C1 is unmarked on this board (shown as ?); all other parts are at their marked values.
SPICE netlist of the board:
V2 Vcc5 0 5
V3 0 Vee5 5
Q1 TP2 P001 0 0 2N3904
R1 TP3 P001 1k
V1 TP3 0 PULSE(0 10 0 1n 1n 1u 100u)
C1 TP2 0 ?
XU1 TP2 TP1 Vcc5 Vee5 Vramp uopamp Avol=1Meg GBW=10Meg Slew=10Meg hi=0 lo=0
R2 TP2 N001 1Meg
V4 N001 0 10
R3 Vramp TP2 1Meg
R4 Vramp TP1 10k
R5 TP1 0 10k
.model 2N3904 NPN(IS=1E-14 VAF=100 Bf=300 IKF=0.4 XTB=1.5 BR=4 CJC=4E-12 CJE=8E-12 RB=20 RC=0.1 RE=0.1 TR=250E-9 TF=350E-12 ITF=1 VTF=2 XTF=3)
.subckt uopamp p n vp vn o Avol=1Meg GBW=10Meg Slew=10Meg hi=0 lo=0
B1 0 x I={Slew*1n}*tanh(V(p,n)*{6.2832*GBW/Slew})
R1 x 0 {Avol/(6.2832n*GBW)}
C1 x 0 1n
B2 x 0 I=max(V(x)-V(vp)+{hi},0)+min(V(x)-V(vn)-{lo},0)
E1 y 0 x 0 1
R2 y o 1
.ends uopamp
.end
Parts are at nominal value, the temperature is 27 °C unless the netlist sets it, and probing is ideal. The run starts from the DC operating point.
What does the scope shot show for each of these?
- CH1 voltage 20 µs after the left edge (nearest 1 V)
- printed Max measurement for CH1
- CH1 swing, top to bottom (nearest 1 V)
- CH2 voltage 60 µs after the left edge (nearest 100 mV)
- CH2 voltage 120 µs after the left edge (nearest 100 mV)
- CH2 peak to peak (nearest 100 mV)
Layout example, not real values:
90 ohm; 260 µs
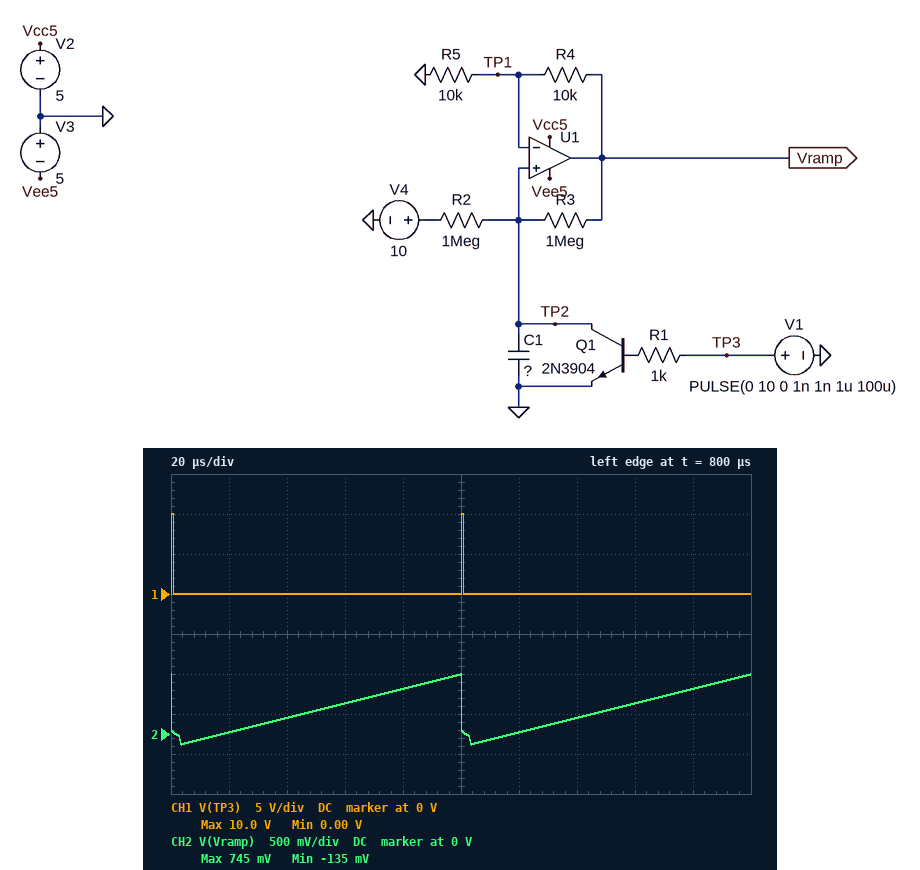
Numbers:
0 V; 10.0 V; 10 V; 400 mV; 0 V; 900 mV
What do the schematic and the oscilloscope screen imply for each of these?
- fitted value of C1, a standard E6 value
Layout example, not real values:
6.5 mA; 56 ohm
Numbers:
2.2 nF
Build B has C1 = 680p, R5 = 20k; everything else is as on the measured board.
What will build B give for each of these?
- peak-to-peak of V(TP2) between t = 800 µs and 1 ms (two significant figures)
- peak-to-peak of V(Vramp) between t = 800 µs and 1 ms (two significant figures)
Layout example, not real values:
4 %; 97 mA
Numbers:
1.4 V; 2.1 V
